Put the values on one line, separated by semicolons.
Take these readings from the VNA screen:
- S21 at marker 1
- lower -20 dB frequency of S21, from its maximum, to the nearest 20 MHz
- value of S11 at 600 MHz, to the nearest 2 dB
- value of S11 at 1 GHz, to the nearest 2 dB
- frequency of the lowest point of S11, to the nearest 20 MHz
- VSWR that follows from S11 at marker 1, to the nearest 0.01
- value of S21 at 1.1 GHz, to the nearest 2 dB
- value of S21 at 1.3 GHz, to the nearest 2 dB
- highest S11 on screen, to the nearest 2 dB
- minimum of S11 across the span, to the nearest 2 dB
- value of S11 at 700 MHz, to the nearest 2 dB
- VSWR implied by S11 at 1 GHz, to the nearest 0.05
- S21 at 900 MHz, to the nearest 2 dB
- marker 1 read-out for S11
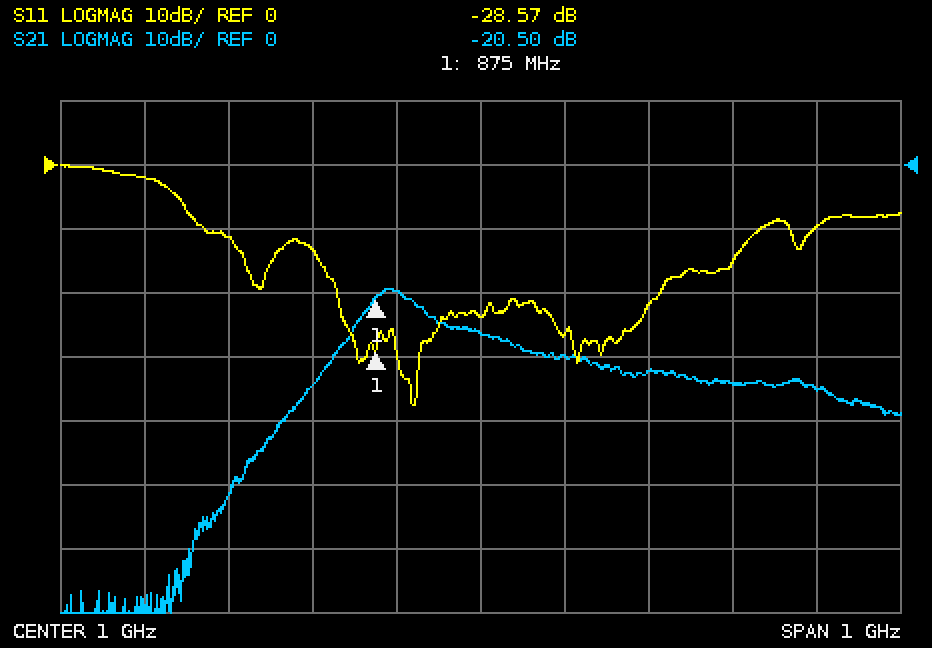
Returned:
-20.50 dB; 760 MHz; -2 dB; -24 dB; 920 MHz; 1.08; -30 dB; -34 dB; 0 dB; -38 dB; -12 dB; 1.15; -20 dB; -28.57 dB
